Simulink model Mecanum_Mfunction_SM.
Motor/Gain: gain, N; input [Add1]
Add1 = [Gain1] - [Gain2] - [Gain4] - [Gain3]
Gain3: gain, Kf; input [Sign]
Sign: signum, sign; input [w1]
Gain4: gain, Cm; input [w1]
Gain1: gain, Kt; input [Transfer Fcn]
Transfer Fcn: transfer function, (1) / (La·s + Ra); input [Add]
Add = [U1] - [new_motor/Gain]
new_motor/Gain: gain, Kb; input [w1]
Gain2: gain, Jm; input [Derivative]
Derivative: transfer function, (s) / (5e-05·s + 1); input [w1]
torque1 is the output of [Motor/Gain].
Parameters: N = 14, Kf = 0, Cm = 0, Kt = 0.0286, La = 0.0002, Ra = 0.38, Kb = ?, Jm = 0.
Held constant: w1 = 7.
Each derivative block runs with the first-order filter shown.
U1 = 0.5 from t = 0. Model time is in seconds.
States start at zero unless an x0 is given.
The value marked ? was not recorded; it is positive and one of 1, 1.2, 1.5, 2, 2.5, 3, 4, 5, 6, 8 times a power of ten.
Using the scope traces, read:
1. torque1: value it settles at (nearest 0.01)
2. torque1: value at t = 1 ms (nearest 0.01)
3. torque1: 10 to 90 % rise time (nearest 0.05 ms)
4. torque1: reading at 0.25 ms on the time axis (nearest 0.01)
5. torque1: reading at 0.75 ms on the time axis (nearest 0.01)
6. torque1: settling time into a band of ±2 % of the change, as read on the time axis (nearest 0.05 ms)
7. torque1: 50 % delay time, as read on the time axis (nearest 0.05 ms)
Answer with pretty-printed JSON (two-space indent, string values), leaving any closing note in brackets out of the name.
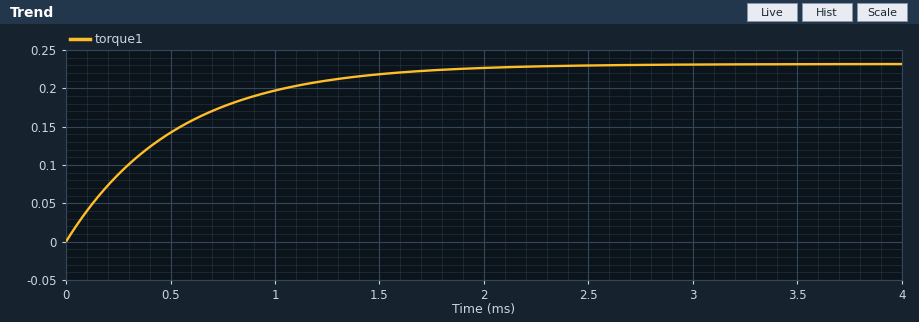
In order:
{
  "torque1: value it settles at": "0.23",
  "torque1: value at t = 1 ms": "0.20",
  "torque1: 10 to 90 % rise time": "1.15 ms",
  "torque1: reading at 0.25 ms on the time axis": "0.09",
  "torque1: reading at 0.75 ms on the time axis": "0.18",
  "torque1: settling time into a band of ±2 % of the change, as read on the time axis": "2.05 ms",
  "torque1: 50 % delay time, as read on the time axis": "0.35 ms"
}
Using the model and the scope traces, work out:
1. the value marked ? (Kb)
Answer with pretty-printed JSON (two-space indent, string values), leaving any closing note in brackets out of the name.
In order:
{
  "the value marked ?": "0.04"
}
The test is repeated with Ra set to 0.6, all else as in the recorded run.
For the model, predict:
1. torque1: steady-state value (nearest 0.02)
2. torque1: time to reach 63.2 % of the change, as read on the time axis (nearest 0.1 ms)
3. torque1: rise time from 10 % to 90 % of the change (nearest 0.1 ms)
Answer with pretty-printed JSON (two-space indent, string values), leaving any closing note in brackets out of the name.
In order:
{
  "torque1: steady-state value": "0.14",
  "torque1: time to reach 63.2 % of the change, as read on the time axis": "0.3 ms",
  "torque1: rise time from 10 % to 90 % of the change": "0.7 ms"
}
